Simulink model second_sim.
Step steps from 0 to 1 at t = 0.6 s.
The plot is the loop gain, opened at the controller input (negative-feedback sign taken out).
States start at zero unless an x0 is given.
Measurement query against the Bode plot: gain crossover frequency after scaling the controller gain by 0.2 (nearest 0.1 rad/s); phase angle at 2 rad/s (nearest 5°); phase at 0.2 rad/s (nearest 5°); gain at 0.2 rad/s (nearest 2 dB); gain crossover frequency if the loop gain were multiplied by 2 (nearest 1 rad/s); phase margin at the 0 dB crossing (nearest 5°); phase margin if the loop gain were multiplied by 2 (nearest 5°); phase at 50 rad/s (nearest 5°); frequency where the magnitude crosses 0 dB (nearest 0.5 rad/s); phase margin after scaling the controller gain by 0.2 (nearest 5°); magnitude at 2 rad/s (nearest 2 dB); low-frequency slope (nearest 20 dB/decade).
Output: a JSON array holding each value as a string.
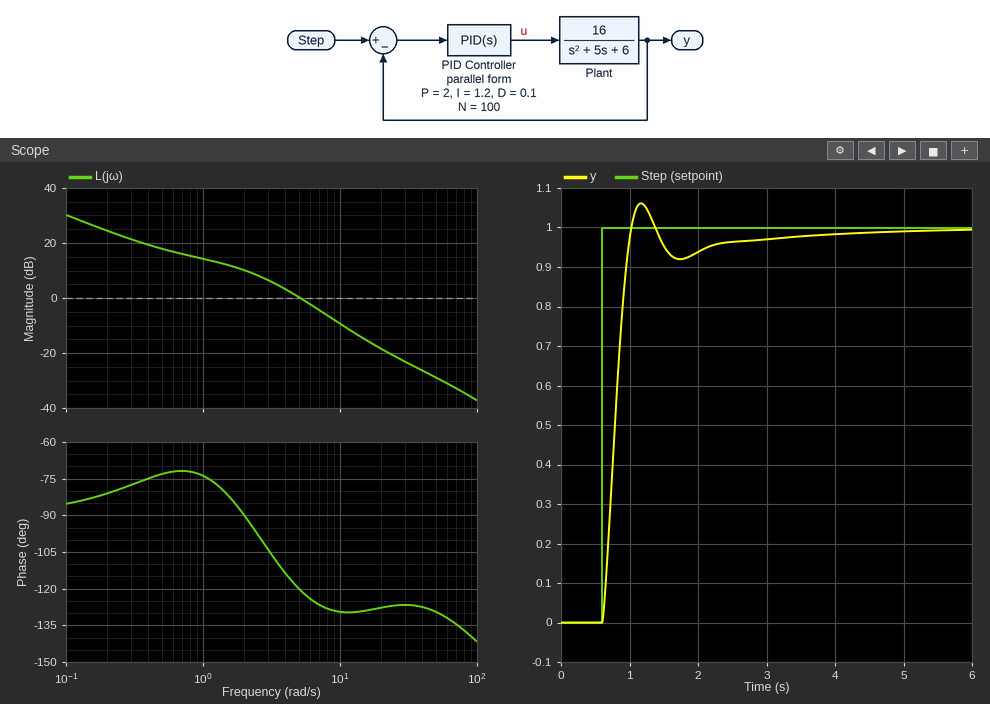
["1.1 rad/s", "-90°", "-80°", "24 dB", "8 rad/s", "60°", "50°", "-130°", "5.0 rad/s", "105°", "10 dB", "-20 dB/decade"]
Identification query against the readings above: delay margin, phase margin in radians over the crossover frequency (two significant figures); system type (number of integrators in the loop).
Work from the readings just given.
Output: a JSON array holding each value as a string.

["0.21 s", "1"]
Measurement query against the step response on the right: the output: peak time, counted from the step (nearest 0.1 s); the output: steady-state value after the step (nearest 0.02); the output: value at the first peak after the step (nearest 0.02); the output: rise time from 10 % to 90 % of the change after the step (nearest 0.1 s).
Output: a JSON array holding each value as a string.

["0.6 s", "1.00", "1.06", "0.3 s"]
